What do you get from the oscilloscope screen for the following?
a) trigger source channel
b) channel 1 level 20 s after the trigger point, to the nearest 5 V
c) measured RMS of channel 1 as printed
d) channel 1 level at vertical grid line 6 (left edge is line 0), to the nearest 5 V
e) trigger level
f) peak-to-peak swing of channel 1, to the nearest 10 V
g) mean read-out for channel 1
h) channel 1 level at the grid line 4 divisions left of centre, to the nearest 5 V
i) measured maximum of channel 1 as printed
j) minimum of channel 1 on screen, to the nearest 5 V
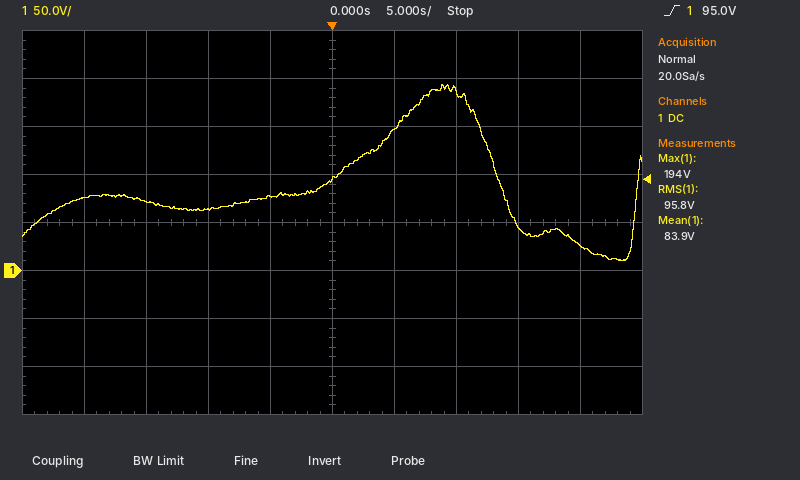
channel 1
25 V
95.8 V
145 V
95.0 V
180 V
83.9 V
75 V
194 V
10 V
